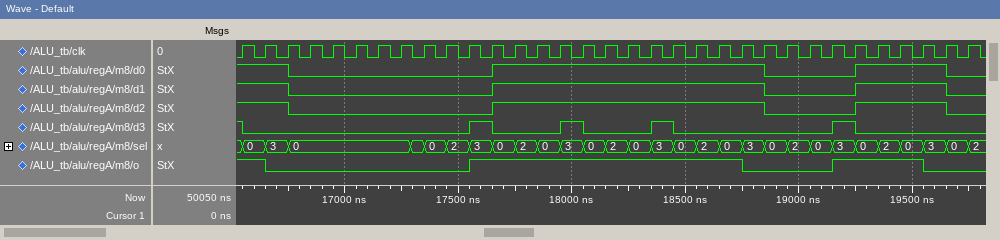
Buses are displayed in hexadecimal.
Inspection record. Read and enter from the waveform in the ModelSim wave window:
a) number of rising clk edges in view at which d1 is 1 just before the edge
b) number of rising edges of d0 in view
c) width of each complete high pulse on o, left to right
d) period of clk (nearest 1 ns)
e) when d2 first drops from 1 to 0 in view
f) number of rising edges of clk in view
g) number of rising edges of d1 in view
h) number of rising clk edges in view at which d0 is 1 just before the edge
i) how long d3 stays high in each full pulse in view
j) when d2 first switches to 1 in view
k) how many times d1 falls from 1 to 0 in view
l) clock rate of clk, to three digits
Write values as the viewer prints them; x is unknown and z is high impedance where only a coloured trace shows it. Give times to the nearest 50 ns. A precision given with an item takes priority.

19
2
1200 ns, 400 ns
100 ns
16750 ns
33
2
19
100 ns, 100 ns, 100 ns, 100 ns
17650 ns
3
10.0 MHz
